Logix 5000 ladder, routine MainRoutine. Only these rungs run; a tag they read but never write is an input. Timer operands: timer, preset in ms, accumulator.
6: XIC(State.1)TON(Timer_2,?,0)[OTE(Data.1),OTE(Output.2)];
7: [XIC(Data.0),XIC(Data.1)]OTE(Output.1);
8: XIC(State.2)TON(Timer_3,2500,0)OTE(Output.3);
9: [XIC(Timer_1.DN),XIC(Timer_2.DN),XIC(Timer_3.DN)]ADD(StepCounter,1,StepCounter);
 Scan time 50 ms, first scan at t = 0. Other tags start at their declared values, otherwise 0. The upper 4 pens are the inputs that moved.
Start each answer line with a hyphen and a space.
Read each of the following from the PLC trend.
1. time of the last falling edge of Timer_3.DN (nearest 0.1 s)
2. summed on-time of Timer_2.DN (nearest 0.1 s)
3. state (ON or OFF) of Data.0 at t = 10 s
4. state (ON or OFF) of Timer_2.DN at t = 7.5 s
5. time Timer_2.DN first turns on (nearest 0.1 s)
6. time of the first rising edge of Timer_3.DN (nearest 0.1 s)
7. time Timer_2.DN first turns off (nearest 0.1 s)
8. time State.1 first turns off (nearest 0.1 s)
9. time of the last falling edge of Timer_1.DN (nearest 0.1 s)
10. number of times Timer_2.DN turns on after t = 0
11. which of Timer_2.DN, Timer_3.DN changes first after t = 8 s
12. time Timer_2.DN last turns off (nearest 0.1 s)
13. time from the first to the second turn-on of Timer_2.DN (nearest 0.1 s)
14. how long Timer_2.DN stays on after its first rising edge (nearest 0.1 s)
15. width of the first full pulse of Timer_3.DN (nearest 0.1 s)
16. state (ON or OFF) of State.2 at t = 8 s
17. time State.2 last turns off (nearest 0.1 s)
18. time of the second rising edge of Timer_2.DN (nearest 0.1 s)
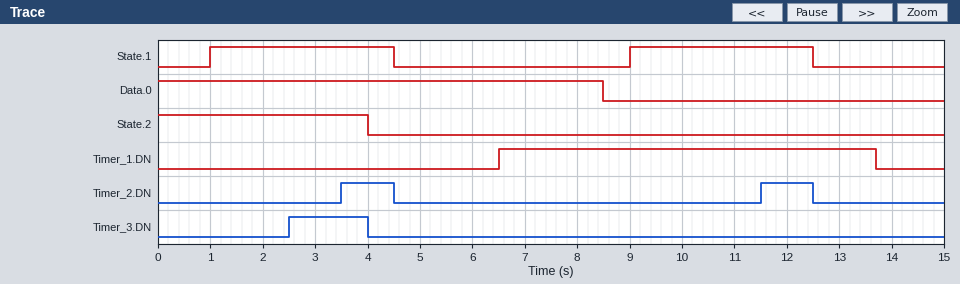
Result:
- 4.0 s
- 2.0 s
- OFF
- OFF
- 3.5 s
- 2.5 s
- 4.5 s
- 4.5 s
- 13.7 s
- 2
- Timer_2.DN
- 12.5 s
- 8.0 s
- 1.0 s
- 1.5 s
- OFF
- 4.0 s
- 11.5 s
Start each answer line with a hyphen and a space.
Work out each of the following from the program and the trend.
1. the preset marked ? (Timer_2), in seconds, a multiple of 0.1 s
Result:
- 2.5 s
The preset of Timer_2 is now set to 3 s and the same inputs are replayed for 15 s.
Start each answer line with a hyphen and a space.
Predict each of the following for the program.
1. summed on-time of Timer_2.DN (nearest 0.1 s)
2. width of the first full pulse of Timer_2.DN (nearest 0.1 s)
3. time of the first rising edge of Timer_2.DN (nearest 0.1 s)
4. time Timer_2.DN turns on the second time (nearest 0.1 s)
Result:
- 1.0 s
- 0.5 s
- 4.0 s
- 12.0 s
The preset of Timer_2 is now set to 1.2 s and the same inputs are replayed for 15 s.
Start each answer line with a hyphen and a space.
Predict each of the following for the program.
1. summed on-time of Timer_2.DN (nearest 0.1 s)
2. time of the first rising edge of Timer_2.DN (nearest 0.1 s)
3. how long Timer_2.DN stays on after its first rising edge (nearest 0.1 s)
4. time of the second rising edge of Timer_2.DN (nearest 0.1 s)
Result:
- 4.6 s
- 2.2 s
- 2.3 s
- 10.2 s
